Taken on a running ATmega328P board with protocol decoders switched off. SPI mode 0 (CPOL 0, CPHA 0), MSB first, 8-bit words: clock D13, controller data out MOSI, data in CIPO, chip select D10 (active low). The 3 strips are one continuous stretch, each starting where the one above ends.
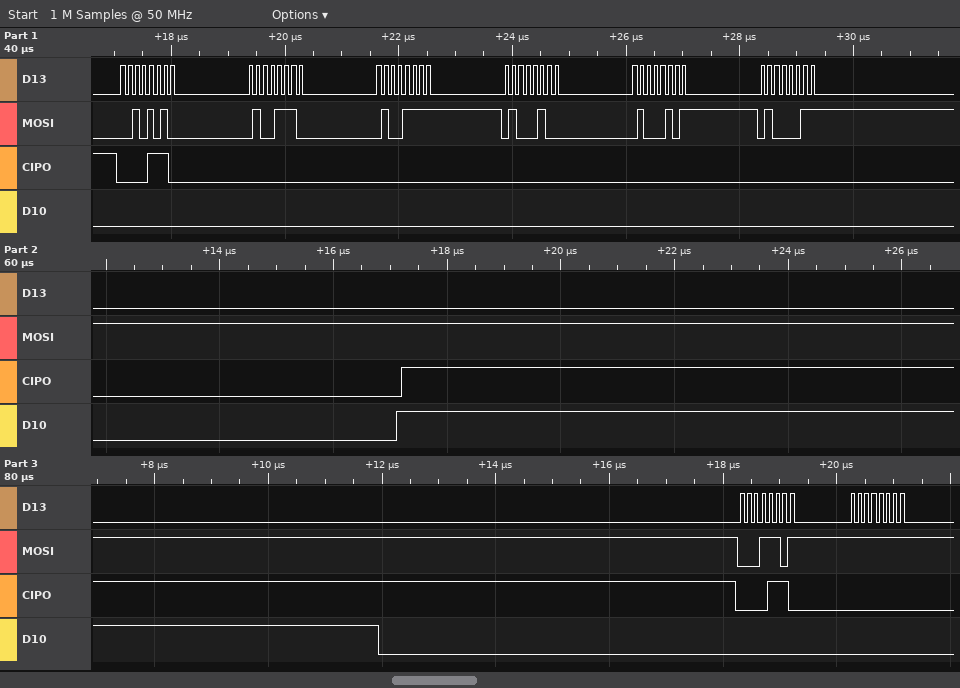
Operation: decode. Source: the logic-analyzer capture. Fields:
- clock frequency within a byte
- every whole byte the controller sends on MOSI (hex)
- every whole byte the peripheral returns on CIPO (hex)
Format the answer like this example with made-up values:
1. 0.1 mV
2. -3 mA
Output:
1. 8 MHz
2. 2A 4E 4F 44 45 43 1D FF
3. 0E 00 00 00 00 00 0E 00
